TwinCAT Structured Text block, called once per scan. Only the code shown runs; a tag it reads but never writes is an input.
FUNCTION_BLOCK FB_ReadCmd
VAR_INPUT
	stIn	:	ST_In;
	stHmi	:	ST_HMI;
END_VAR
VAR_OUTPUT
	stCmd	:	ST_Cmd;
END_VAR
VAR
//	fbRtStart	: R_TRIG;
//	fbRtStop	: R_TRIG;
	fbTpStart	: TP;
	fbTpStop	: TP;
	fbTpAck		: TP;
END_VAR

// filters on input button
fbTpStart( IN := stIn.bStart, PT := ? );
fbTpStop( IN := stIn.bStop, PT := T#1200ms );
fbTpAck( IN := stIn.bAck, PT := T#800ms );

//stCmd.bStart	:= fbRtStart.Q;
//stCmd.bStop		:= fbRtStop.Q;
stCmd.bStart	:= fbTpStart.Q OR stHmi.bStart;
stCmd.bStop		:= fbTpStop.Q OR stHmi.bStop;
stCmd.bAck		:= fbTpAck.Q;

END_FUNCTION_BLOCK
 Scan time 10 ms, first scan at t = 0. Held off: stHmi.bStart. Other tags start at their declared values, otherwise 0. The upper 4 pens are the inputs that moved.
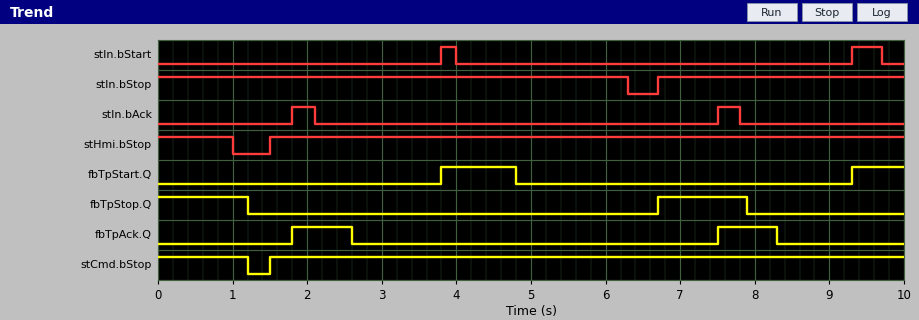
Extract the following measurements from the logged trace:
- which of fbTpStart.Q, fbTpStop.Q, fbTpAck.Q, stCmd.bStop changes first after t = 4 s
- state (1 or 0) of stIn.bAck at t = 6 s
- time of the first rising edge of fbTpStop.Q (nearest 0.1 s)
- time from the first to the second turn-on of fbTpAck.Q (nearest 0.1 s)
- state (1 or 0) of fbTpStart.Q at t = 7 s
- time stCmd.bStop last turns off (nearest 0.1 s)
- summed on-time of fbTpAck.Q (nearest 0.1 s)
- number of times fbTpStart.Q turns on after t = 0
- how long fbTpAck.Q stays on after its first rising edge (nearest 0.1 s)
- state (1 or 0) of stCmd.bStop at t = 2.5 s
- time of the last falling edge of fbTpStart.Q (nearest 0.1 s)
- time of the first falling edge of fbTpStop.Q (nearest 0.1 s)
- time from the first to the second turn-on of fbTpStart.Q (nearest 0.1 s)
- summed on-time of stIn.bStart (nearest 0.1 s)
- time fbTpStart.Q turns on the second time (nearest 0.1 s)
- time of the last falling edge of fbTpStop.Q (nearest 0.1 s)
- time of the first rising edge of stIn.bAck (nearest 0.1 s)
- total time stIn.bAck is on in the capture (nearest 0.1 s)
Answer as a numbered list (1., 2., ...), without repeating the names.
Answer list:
1. fbTpStart.Q
2. 0
3. 6.7 s
4. 5.7 s
5. 0
6. 1.2 s
7. 1.6 s
8. 2
9. 0.8 s
10. 1
11. 4.8 s
12. 1.2 s
13. 5.5 s
14. 0.6 s
15. 9.3 s
16. 7.9 s
17. 1.8 s
18. 0.6 s
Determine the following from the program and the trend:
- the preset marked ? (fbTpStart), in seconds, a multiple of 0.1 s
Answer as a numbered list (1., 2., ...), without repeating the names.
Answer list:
1. 1.0 s
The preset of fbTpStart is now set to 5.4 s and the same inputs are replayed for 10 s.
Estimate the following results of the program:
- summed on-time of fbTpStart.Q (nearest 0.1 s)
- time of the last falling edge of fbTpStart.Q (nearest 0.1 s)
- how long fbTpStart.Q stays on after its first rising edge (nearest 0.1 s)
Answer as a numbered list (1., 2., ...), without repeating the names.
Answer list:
1. 6.1 s
2. 9.2 s
3. 5.4 s
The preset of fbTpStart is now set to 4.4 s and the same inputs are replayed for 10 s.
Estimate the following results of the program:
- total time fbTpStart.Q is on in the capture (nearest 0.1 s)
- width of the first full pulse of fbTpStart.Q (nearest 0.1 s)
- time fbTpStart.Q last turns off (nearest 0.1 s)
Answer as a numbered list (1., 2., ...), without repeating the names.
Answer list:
1. 5.1 s
2. 4.4 s
3. 8.2 s
